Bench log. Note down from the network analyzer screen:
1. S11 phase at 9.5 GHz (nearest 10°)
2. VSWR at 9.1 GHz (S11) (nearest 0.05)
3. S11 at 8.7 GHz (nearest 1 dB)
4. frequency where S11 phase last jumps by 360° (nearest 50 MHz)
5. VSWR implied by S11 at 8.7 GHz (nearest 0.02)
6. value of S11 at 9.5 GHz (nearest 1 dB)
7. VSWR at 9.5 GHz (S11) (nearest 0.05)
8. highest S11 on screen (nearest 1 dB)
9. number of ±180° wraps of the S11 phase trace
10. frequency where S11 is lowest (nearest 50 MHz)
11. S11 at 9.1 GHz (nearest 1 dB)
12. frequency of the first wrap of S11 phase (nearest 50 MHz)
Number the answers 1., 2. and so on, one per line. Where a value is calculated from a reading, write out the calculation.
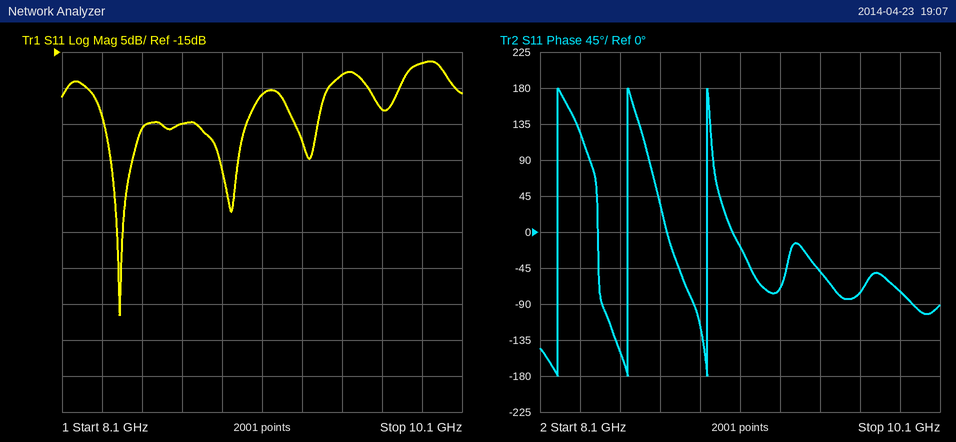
1. -50°
2. |Γ| = 10^(-21/20) = 0.0891; VSWR = (1 + 0.0891)/(1 − 0.0891) ≈ 1.20
3. -25 dB
4. 8.95 GHz
5. |Γ| = 10^(-25/20) = 0.0562; VSWR = (1 + 0.0562)/(1 − 0.0562) ≈ 1.12
6. -18 dB
7. |Γ| = 10^(-18/20) = 0.1259; VSWR = (1 + 0.1259)/(1 − 0.1259) ≈ 1.29, so 1.30 to the nearest 0.05
8. -16 dB
9. 3
10. 8.40 GHz
11. -21 dB
12. 8.20 GHz
